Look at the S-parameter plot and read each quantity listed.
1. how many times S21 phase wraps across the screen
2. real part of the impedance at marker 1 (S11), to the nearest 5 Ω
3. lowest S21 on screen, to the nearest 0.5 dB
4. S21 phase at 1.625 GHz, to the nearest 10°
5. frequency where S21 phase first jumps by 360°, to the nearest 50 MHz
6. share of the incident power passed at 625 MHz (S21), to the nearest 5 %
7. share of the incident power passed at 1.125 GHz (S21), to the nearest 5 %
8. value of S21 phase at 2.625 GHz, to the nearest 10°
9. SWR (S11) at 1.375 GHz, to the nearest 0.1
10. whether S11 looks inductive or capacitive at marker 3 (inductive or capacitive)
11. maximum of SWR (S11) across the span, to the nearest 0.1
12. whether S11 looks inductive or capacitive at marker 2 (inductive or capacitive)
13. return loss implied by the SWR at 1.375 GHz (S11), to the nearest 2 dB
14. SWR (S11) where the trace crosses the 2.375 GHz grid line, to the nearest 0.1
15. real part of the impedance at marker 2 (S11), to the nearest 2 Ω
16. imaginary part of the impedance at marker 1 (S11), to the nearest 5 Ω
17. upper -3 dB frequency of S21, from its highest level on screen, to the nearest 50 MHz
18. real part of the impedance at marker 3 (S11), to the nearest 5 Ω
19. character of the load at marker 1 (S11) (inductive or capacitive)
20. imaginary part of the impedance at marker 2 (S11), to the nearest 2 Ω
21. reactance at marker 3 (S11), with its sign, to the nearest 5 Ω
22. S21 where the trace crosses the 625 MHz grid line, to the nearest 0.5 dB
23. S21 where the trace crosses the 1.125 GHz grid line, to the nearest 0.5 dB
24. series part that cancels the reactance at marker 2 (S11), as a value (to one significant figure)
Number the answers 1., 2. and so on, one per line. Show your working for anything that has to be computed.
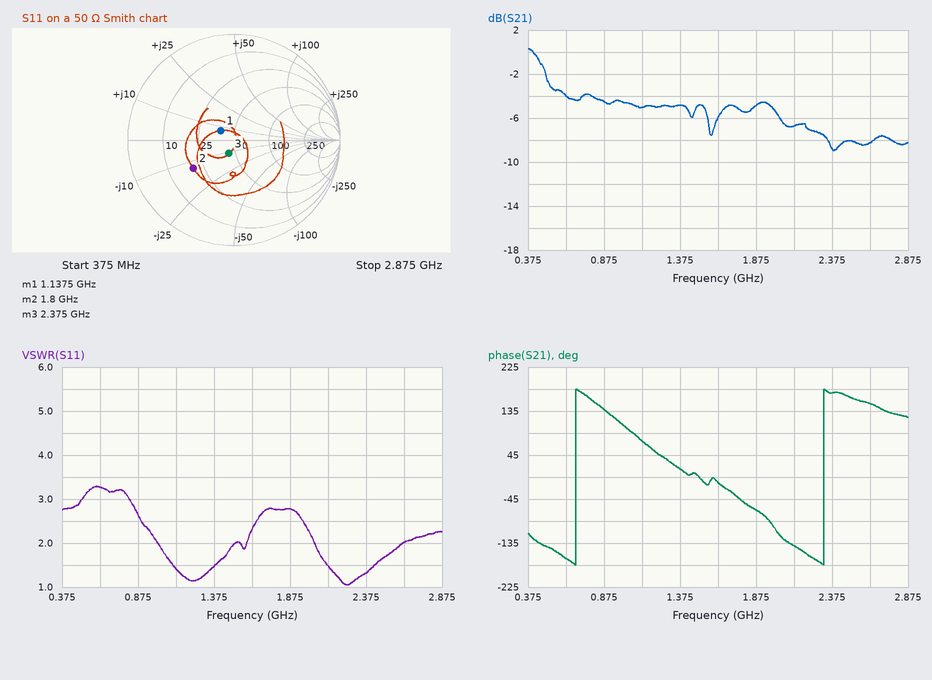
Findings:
1. 2
2. 40 Ω
3. -9.0 dB
4. -10°
5. 700 MHz
6. 10^(-4/10) ≈ 40 %
7. 10^(-5/10) ≈ 31.6 %, so 30 % to the nearest 5 %
8. 150°
9. 1.5
10. capacitive
11. 3.3
12. capacitive
13. −20 log10((1.5 − 1)/(1.5 + 1)) ≈ 14 dB
14. 1.3
15. 20 Ω
16. +5 Ω
17. 500 MHz
18. 45 Ω
19. inductive
20. -14 Ω
21. -10 Ω
22. -4.0 dB
23. -5.0 dB
24. L = 14 Ω/(2π × 1.8 GHz) ≈ 1 nH
